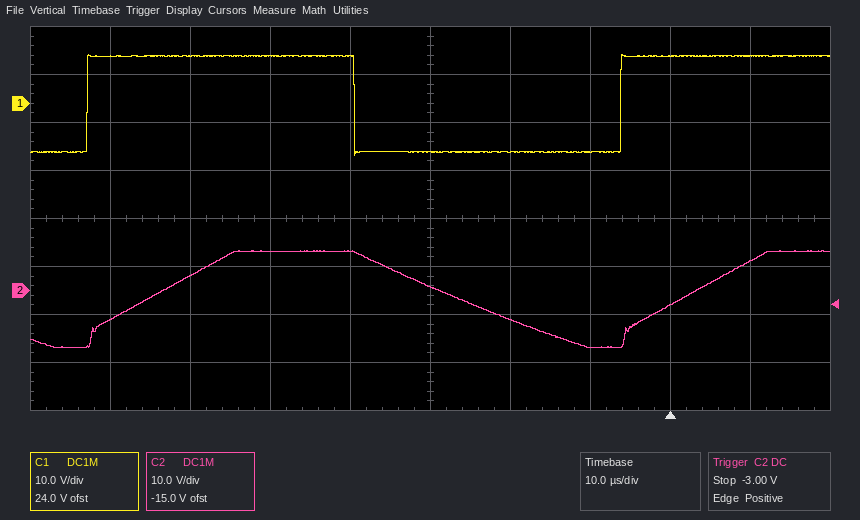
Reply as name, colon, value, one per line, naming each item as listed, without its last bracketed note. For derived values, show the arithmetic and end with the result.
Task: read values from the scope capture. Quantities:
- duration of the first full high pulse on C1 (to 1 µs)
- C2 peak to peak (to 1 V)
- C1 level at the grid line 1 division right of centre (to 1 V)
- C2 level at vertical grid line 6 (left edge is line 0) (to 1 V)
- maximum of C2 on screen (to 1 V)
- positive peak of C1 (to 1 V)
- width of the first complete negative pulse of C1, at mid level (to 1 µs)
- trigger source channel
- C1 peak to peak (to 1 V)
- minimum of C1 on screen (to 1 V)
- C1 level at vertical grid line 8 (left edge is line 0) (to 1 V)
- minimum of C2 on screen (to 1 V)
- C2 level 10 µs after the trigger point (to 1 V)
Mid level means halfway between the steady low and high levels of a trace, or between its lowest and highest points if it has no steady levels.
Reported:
duration of the first full high pulse on C1: 33 µs
C2 peak to peak: 8 V − (-12 V) = 20 V
C1 level at the grid line 1 division right of centre: -10 V
C2 level at vertical grid line 6 (left edge is line 0): -6 V
maximum of C2 on screen: 8 V
positive peak of C1: 10 V
width of the first complete negative pulse of C1, at mid level: 33 µs
trigger source channel: C2
C1 peak to peak: 10 V − (-11 V) = 21 V
minimum of C1 on screen: -11 V
C1 level at vertical grid line 8 (left edge is line 0): 10 V
minimum of C2 on screen: -12 V
C2 level 10 µs after the trigger point: 6 V
